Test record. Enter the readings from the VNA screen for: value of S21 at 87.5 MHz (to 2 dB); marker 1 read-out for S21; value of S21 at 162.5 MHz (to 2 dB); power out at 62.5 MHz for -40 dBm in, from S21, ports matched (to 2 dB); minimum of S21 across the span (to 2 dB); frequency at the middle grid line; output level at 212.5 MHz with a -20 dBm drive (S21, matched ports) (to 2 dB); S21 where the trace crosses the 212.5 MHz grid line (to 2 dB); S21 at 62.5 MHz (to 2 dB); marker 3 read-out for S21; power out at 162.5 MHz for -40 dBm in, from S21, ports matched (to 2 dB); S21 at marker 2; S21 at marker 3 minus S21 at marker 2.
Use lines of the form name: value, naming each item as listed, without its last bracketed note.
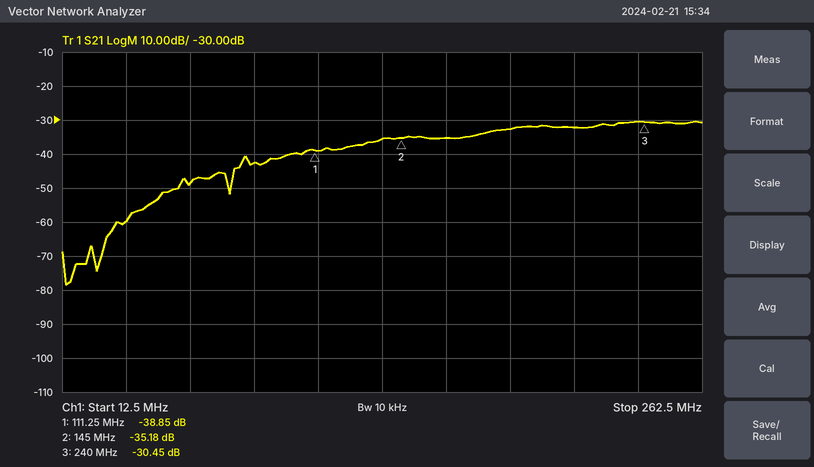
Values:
value of S21 at 87.5 MHz: -42 dB
marker 1 read-out for S21: -38.85 dB
value of S21 at 162.5 MHz: -36 dB
power out at 62.5 MHz for -40 dBm in, from S21, ports matched: -88 dBm
minimum of S21 across the span: -78 dB
frequency at the middle grid line: 137.5 MHz
output level at 212.5 MHz with a -20 dBm drive (S21, matched ports): -52 dBm
S21 where the trace crosses the 212.5 MHz grid line: -32 dB
S21 at 62.5 MHz: -48 dB
marker 3 read-out for S21: -30.45 dB
power out at 162.5 MHz for -40 dBm in, from S21, ports matched: -76 dBm
S21 at marker 2: -35.18 dB
S21 at marker 3 minus S21 at marker 2: 4.73 dB
